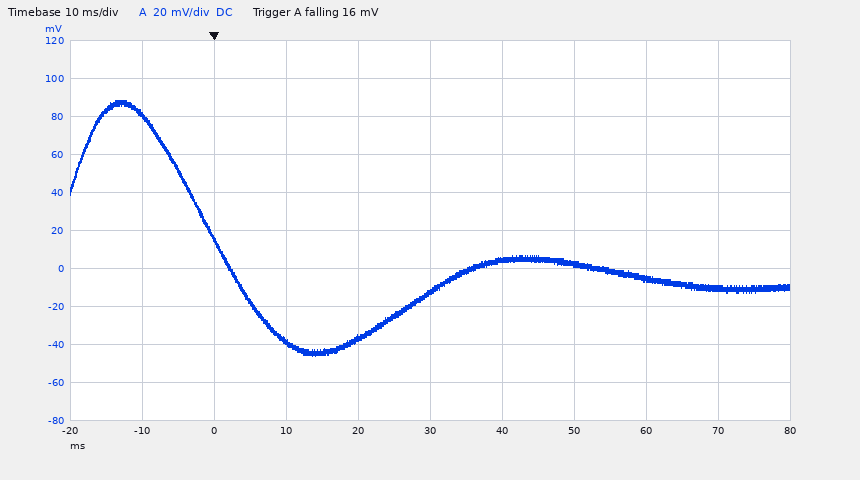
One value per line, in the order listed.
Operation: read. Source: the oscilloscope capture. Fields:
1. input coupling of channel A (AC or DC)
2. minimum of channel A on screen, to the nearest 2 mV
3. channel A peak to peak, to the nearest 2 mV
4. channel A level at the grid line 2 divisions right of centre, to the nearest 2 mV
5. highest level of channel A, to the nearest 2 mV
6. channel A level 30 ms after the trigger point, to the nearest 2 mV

DC
-46 mV
134 mV
2 mV
88 mV
-12 mV
